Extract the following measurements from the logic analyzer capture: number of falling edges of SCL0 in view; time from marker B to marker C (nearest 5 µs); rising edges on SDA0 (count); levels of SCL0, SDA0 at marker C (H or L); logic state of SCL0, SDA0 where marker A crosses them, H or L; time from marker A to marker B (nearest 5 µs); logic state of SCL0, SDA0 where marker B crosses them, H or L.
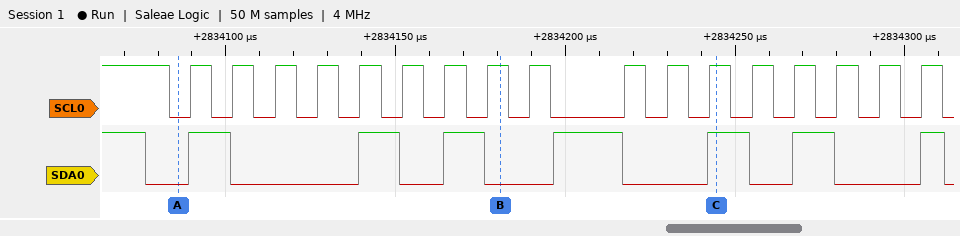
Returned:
18
65 µs
7
SCL0=H, SDA0=H
SCL0=L, SDA0=L
95 µs
SCL0=H, SDA0=L
